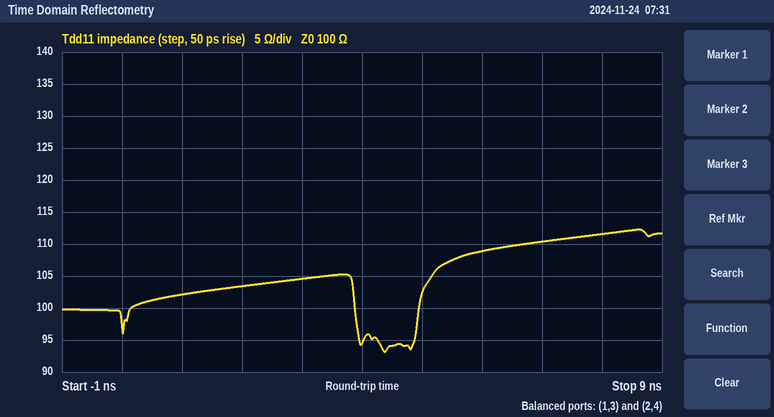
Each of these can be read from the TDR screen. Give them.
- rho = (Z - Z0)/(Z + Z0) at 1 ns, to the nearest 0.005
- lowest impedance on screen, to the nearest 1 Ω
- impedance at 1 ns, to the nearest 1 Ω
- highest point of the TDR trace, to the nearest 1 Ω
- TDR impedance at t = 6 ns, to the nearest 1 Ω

+0.010
93 Ω
102 Ω
112 Ω
109 Ω
